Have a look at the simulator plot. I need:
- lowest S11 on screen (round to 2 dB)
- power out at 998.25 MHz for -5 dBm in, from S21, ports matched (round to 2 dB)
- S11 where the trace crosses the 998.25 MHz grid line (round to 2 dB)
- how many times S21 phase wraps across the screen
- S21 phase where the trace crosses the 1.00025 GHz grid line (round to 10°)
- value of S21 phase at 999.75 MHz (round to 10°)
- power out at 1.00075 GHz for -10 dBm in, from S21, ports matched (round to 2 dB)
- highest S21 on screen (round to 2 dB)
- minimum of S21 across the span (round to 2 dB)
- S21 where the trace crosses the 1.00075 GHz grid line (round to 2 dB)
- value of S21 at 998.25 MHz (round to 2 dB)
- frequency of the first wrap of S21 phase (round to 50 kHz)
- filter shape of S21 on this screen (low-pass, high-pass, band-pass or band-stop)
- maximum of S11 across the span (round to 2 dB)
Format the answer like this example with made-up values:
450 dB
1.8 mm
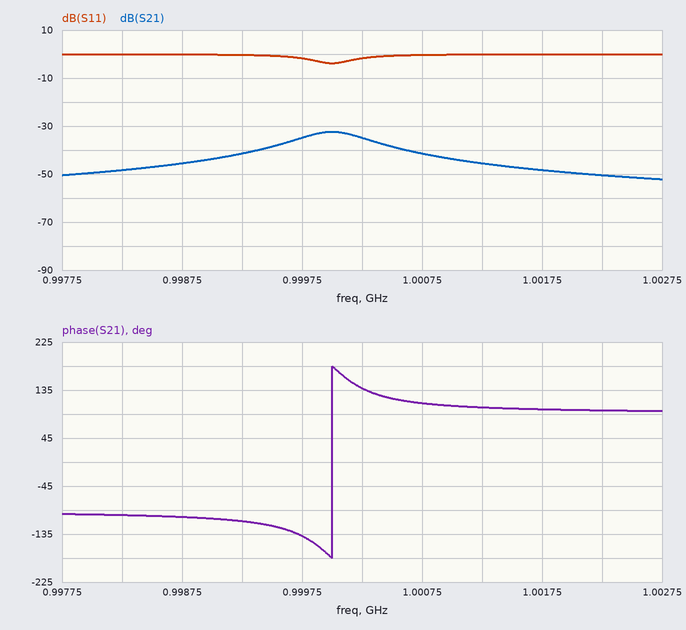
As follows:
-4 dB
-54 dBm
0 dB
1
140°
-140°
-52 dBm
-32 dB
-52 dB
-42 dB
-48 dB
1.00000 GHz
band-pass
0 dB
